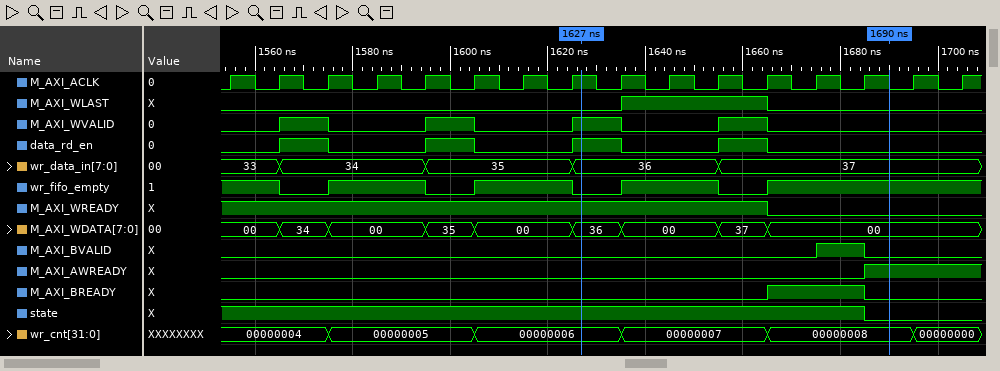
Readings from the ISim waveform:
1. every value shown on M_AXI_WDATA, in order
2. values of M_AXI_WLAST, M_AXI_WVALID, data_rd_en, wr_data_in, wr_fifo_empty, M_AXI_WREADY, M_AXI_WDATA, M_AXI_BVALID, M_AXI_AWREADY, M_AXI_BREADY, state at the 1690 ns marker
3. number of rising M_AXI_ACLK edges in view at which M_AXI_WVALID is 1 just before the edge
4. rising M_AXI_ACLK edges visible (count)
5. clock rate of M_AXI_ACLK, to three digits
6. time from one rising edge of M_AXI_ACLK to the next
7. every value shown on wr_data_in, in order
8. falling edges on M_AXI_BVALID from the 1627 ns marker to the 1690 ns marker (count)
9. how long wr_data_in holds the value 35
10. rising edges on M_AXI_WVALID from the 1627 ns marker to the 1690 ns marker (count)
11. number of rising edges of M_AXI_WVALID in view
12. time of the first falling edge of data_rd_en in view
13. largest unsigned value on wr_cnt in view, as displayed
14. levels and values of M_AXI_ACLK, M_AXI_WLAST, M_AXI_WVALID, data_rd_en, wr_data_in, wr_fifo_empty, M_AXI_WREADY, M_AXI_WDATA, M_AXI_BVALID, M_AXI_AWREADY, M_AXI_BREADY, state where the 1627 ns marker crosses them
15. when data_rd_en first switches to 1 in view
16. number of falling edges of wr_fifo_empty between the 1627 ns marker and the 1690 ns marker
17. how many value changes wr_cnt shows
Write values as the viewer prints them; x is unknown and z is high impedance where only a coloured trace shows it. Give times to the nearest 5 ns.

00, 34, 00, 35, 00, 36, 00, 37, 00
M_AXI_WLAST=0, M_AXI_WVALID=0, data_rd_en=0, wr_data_in=37, wr_fifo_empty=1, M_AXI_WREADY=0, M_AXI_WDATA=00, M_AXI_BVALID=0, M_AXI_AWREADY=1, M_AXI_BREADY=0, state=0
4
16
100 MHz
10 ns
33, 34, 35, 36, 37
1
30 ns
1
4
1575 ns
00000008
M_AXI_ACLK=1, M_AXI_WLAST=0, M_AXI_WVALID=1, data_rd_en=1, wr_data_in=36, wr_fifo_empty=0, M_AXI_WREADY=1, M_AXI_WDATA=36, M_AXI_BVALID=0, M_AXI_AWREADY=0, M_AXI_BREADY=0, state=1
1565 ns
1
5
